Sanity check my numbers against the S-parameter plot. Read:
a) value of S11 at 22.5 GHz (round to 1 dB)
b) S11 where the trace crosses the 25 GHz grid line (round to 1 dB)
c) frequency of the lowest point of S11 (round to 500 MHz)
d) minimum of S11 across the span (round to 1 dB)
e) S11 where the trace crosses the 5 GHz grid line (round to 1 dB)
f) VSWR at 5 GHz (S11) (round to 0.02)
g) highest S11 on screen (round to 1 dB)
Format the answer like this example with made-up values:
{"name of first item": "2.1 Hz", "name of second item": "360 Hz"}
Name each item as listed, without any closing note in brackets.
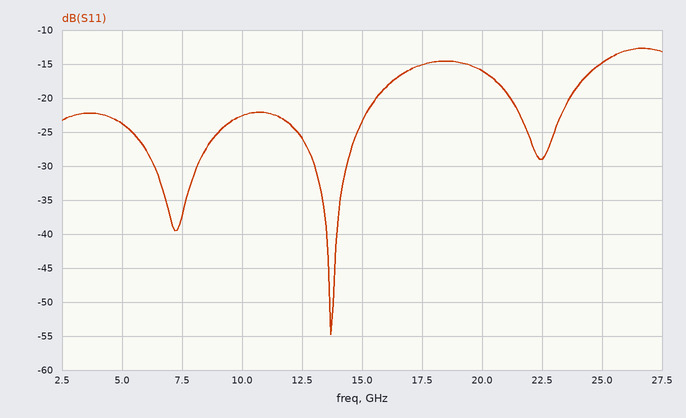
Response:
{"value of S11 at 22.5 GHz": "-29 dB", "S11 where the trace crosses the 25 GHz grid line": "-15 dB", "frequency of the lowest point of S11": "13.5 GHz", "minimum of S11 across the span": "-55 dB", "S11 where the trace crosses the 5 GHz grid line": "-24 dB", "VSWR at 5 GHz (S11)": "1.14", "highest S11 on screen": "-13 dB"}
